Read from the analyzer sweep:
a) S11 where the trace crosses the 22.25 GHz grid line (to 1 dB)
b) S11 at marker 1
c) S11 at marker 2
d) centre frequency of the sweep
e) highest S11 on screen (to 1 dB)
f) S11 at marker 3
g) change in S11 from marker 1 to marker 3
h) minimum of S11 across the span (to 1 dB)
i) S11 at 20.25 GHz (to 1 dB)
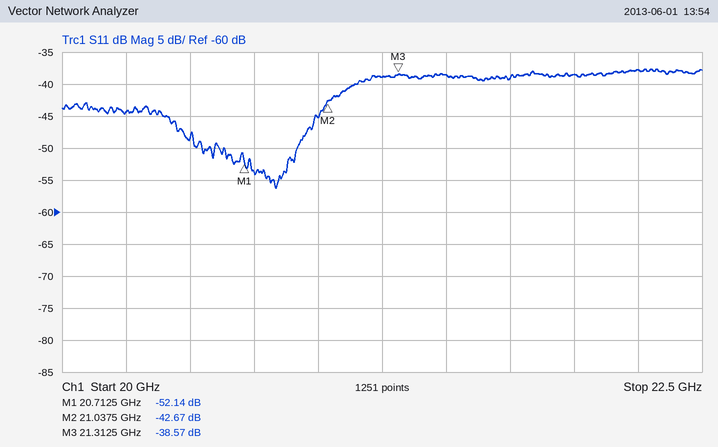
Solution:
-38 dB
-52.14 dB
-42.67 dB
21.25 GHz
-38 dB
-38.57 dB
13.57 dB
-56 dB
-44 dB
